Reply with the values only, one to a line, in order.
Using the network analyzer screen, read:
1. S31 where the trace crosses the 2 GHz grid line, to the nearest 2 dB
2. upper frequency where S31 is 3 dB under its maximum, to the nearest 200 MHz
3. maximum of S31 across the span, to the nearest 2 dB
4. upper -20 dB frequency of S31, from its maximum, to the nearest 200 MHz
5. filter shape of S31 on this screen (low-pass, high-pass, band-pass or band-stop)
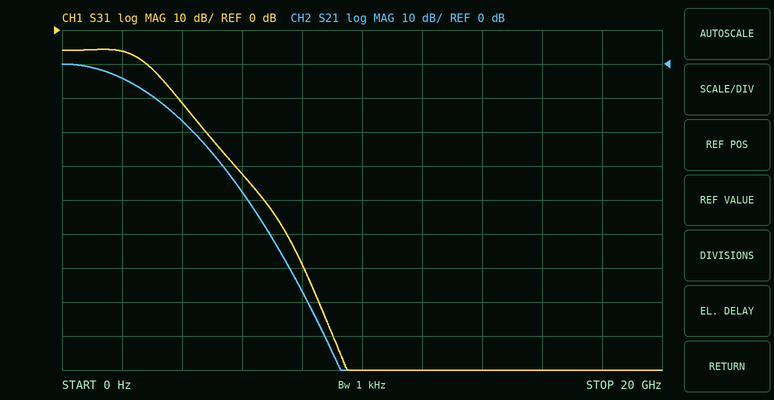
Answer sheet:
-6 dB
2.6 GHz
-6 dB
4.4 GHz
low-pass
